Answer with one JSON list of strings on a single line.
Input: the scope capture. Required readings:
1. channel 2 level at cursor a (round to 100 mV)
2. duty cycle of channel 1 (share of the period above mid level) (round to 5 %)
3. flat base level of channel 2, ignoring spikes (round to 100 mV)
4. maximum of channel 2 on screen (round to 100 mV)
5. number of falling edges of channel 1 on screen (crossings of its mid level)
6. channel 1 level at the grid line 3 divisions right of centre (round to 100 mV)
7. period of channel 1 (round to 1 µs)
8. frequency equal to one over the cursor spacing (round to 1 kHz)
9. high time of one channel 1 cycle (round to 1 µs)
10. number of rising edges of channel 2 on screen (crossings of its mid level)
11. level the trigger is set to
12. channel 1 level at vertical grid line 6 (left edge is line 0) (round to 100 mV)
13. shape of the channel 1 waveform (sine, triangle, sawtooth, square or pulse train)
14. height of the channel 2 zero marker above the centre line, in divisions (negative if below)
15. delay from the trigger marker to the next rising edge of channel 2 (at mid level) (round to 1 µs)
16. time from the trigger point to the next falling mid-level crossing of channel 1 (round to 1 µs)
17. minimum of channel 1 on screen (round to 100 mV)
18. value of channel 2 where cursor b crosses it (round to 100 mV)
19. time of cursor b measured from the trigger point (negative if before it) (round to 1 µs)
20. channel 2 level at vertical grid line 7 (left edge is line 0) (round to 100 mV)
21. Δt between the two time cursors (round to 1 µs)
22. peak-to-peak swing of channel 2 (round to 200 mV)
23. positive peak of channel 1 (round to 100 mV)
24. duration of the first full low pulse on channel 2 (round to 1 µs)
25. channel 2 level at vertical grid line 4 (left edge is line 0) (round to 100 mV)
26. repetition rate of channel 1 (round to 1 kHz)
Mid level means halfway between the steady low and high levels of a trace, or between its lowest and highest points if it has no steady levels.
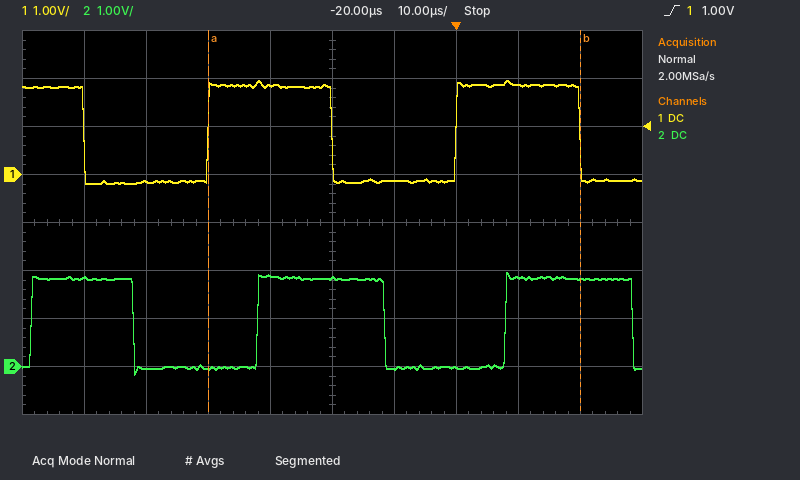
["0.0 V", "50 %", "0.0 V", "2.0 V", "3", "1.9 V", "40 µs", "17 kHz", "20 µs", "3", "1.00 V", "-100 mV", "square", "-3.0 div", "8 µs", "20 µs", "-200 mV", "1.8 V", "+20 µs", "0.0 V", "60 µs", "2.2 V", "2.0 V", "20 µs", "1.9 V", "25 kHz"]
